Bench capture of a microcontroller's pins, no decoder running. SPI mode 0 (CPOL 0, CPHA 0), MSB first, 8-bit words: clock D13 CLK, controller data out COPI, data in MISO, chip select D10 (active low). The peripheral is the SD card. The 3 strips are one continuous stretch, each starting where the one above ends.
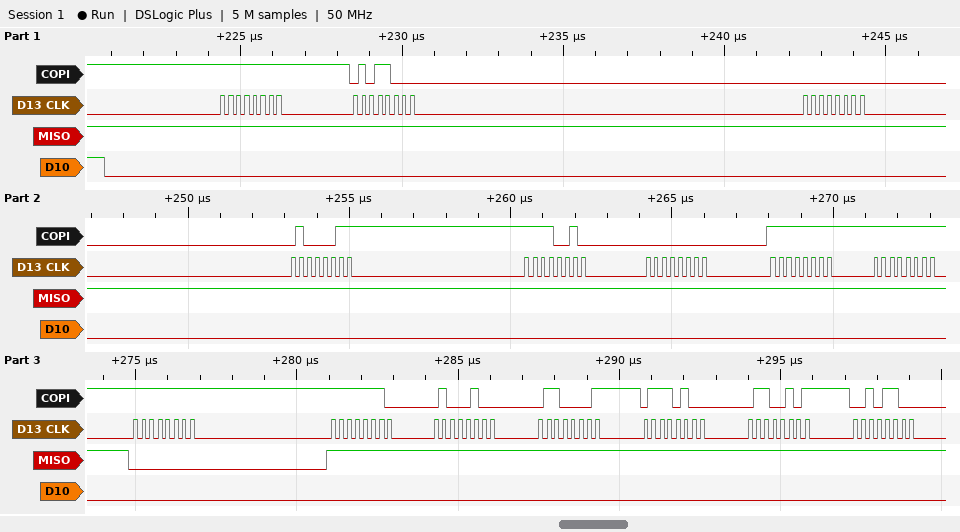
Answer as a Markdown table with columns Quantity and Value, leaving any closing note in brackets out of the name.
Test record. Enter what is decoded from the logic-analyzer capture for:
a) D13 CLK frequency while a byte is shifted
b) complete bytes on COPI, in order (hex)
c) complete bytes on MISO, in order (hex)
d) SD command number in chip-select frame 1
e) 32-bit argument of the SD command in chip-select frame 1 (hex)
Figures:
| Quantity | Value |
|---|---|
| D13 CLK frequency while a byte is shifted | 4 MHz |
| complete bytes on COPI, in order | 0xFF 0x58 0x00 0x43 0xF2 0x00 0xFF 0xFF 0xFF 0xFE 0x44 0x61 0x74 0x65 0x2C |
| complete bytes on MISO, in order | 0xFF 0xFF 0xFF 0xFF 0xFF 0xFF 0xFF 0xFF 0x00 0xFF 0xFF 0xFF 0xFF 0xFF 0xFF |
| SD command number in chip-select frame 1 | CMD24 |
| 32-bit argument of the SD command in chip-select frame 1 | 0x0043F200 |
